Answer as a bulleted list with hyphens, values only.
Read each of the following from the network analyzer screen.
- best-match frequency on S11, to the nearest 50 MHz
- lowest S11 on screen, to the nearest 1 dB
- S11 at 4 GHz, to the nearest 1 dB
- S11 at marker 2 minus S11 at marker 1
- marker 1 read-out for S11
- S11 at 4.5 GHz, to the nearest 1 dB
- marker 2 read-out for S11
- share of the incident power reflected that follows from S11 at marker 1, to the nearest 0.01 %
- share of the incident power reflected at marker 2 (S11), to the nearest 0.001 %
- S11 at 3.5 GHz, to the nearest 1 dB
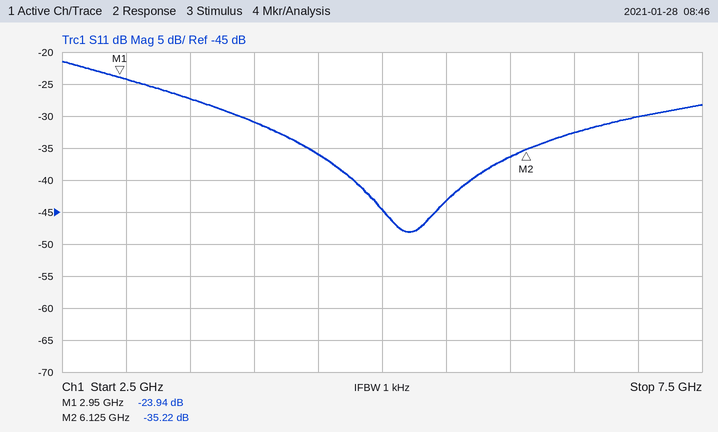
- 5.20 GHz
- -48 dB
- -31 dB
- -11.28 dB
- -23.94 dB
- -36 dB
- -35.22 dB
- 0.40 %
- 0.030 %
- -27 dB
